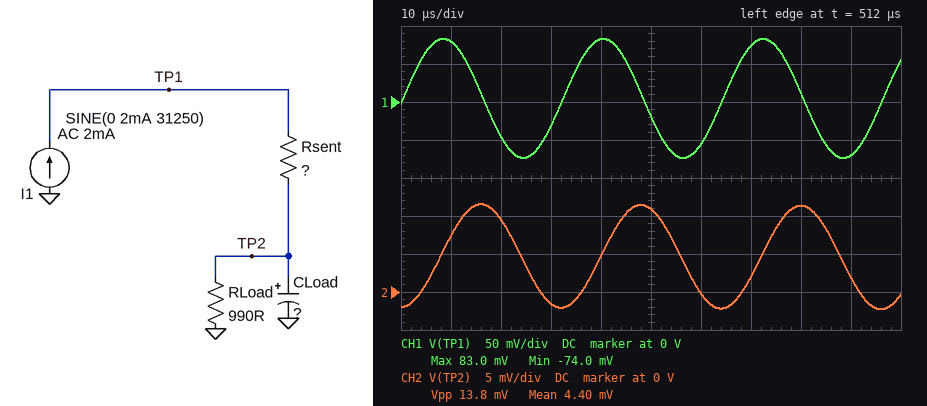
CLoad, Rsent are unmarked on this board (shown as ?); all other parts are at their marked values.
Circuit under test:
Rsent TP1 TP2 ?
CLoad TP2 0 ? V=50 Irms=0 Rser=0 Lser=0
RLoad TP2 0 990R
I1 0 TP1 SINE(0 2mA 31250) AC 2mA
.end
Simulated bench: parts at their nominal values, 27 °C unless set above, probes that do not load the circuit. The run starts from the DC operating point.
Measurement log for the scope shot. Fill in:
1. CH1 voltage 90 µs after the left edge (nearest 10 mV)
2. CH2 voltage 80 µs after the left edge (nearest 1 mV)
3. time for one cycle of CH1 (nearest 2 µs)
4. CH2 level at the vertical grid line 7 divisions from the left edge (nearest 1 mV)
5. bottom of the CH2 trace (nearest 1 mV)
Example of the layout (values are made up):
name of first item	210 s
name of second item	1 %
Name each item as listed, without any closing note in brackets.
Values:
CH1 voltage 90 µs after the left edge	-70 mV
CH2 voltage 80 µs after the left edge	11 mV
time for one cycle of CH1	32 µs
CH2 level at the vertical grid line 7 divisions from the left edge	2 mV
bottom of the CH2 trace	-2 mV
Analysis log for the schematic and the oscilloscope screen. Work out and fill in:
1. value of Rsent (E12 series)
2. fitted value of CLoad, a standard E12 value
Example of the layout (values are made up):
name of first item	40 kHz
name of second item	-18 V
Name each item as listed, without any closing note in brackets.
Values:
value of Rsent	39 Ω
fitted value of CLoad, a standard E12 value	1.5 µF
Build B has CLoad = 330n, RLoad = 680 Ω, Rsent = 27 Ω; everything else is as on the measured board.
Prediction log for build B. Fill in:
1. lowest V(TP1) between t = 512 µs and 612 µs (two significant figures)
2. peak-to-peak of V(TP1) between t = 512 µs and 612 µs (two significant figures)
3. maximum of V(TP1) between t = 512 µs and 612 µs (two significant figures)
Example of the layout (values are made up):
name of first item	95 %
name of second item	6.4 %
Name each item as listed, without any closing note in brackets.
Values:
lowest V(TP1) between t = 512 µs and 612 µs	-61 mV
peak-to-peak of V(TP1) between t = 512 µs and 612 µs	130 mV
maximum of V(TP1) between t = 512 µs and 612 µs	66 mV
